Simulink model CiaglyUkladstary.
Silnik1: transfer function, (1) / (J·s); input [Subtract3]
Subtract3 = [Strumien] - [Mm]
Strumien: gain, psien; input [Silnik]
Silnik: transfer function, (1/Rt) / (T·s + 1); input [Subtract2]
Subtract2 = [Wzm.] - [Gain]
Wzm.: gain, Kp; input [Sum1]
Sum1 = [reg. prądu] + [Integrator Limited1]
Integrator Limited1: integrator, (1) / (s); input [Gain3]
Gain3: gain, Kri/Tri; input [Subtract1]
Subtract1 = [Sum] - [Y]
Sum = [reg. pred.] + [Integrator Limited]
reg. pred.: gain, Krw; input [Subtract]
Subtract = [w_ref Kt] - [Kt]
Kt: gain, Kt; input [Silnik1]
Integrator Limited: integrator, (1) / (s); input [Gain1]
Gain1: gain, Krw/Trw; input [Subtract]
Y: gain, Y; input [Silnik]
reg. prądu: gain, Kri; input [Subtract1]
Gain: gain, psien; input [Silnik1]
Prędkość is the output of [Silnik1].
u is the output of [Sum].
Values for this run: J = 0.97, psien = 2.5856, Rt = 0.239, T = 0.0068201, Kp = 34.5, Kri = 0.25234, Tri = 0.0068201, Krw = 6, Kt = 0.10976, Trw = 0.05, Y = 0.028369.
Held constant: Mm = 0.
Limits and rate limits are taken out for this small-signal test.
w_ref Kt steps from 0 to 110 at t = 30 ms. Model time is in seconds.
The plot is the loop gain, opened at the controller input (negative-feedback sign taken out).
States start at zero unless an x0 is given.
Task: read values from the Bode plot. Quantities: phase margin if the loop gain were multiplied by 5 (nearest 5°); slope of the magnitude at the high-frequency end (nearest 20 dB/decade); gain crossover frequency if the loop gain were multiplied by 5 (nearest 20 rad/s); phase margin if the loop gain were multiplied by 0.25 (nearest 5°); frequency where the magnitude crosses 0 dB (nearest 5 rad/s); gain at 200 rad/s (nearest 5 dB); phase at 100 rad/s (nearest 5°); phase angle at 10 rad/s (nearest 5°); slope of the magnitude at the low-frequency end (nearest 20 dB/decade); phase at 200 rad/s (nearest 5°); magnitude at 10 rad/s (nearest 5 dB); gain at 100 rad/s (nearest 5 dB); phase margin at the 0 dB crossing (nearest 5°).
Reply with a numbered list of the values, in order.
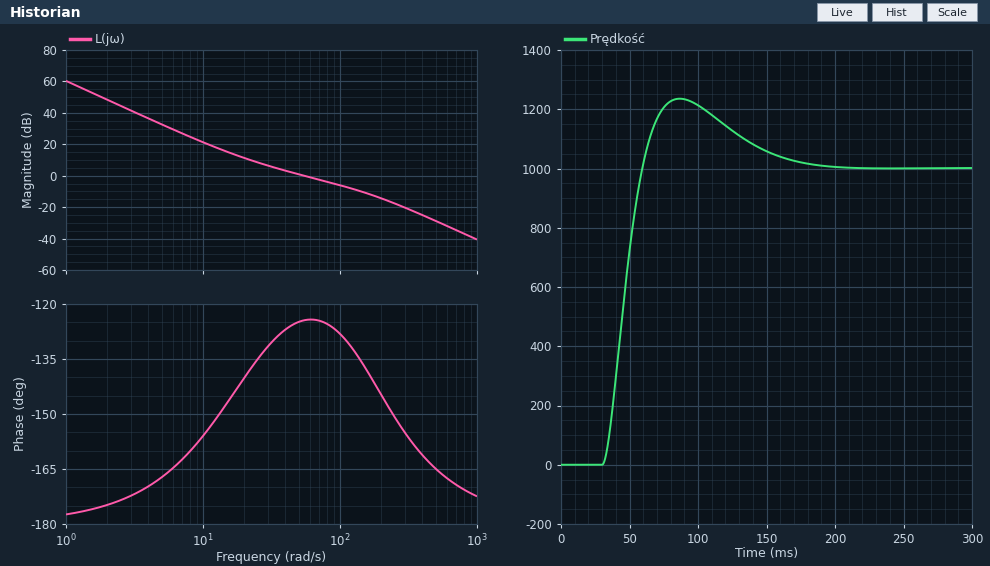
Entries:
1. 35°
2. -40 dB/decade
3. 200 rad/s
4. 40°
5. 55 rad/s
6. -15 dB
7. -130°
8. -155°
9. -40 dB/decade
10. -145°
11. 20 dB
12. -5 dB
13. 55°
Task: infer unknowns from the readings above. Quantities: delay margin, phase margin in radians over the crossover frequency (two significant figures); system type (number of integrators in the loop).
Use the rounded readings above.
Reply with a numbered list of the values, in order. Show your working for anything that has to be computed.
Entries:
1. 55 × π / 180 / 55 = 0.017 s
2. 2
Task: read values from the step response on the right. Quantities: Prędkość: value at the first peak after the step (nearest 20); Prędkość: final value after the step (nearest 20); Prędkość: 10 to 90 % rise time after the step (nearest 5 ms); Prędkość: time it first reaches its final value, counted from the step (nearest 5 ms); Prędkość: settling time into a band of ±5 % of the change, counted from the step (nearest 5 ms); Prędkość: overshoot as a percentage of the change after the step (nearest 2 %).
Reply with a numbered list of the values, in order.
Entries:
1. 1240
2. 1000
3. 20 ms
4. 30 ms
5. 125 ms
6. 24 %
